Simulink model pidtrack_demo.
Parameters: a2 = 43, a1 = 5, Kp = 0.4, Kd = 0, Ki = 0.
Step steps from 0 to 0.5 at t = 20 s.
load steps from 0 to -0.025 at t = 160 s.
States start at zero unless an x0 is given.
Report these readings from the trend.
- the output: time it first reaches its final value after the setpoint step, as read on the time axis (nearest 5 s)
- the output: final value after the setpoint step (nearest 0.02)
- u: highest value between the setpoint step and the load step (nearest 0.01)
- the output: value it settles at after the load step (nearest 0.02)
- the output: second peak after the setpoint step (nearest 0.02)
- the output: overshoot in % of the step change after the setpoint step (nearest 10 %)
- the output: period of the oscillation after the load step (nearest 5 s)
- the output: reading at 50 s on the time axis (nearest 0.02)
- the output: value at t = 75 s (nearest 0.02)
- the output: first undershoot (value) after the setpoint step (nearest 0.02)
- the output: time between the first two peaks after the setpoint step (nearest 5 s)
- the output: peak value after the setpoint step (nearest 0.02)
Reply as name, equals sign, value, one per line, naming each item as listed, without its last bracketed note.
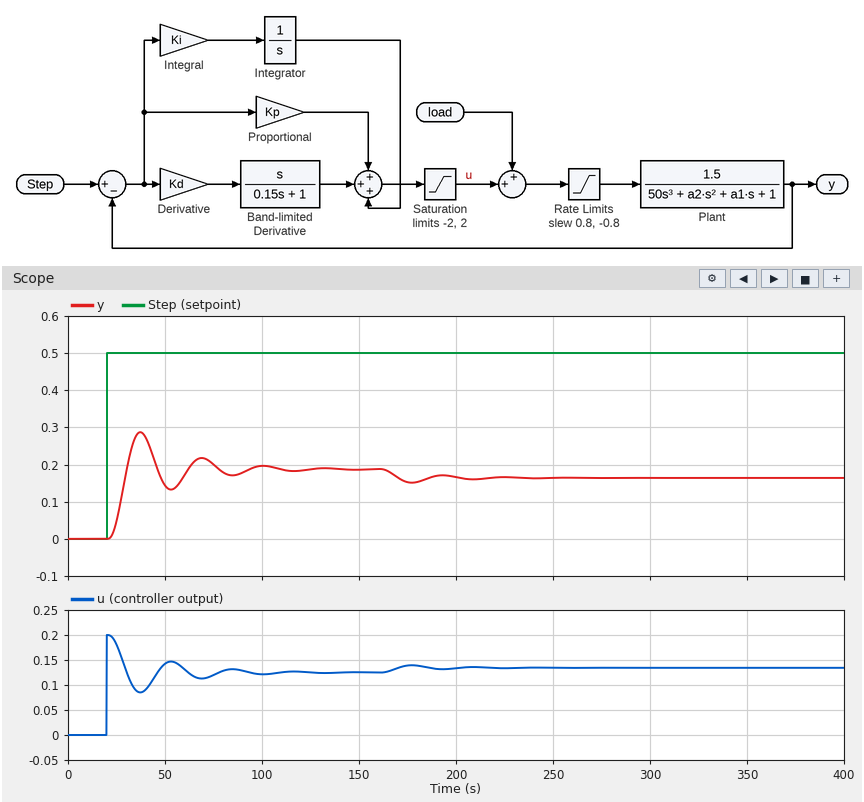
the output: time it first reaches its final value after the setpoint step, as read on the time axis = 30 s
the output: final value after the setpoint step = 0.18
u: highest value between the setpoint step and the load step = 0.20
the output: value it settles at after the load step = 0.16
the output: second peak after the setpoint step = 0.22
the output: overshoot in % of the step change after the setpoint step = 50 %
the output: period of the oscillation after the load step = 30 s
the output: reading at 50 s on the time axis = 0.14
the output: value at t = 75 s = 0.20
the output: first undershoot (value) after the setpoint step = 0.14
the output: time between the first two peaks after the setpoint step = 30 s
the output: peak value after the setpoint step = 0.28
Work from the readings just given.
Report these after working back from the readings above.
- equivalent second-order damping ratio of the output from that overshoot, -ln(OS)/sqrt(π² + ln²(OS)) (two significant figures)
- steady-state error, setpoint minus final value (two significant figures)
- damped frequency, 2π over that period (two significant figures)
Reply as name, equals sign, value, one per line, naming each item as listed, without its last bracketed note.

equivalent second-order damping ratio of the output from that overshoot, -ln(OS)/sqrt(π² + ln²(OS)) = 0.22
steady-state error, setpoint minus final value = 0.32
damped frequency, 2π over that period = 0.21 rad/s
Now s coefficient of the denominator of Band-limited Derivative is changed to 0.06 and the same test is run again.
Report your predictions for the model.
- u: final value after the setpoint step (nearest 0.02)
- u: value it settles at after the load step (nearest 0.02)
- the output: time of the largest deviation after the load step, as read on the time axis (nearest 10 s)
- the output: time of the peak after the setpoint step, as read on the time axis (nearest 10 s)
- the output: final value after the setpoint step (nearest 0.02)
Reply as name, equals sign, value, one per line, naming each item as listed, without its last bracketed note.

u: final value after the setpoint step = 0.12
u: value it settles at after the load step = 0.14
the output: time of the largest deviation after the load step, as read on the time axis = 180 s
the output: time of the peak after the setpoint step, as read on the time axis = 40 s
the output: final value after the setpoint step = 0.18
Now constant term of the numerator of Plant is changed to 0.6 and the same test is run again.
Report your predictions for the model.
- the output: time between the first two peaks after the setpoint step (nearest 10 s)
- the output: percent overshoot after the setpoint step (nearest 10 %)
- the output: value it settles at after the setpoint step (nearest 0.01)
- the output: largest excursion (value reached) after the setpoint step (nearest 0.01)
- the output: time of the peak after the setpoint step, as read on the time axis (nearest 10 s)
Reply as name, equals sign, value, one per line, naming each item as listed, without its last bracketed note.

the output: time between the first two peaks after the setpoint step = 40 s
the output: percent overshoot after the setpoint step = 40 %
the output: value it settles at after the setpoint step = 0.10
the output: largest excursion (value reached) after the setpoint step = 0.14
the output: time of the peak after the setpoint step, as read on the time axis = 40 s
